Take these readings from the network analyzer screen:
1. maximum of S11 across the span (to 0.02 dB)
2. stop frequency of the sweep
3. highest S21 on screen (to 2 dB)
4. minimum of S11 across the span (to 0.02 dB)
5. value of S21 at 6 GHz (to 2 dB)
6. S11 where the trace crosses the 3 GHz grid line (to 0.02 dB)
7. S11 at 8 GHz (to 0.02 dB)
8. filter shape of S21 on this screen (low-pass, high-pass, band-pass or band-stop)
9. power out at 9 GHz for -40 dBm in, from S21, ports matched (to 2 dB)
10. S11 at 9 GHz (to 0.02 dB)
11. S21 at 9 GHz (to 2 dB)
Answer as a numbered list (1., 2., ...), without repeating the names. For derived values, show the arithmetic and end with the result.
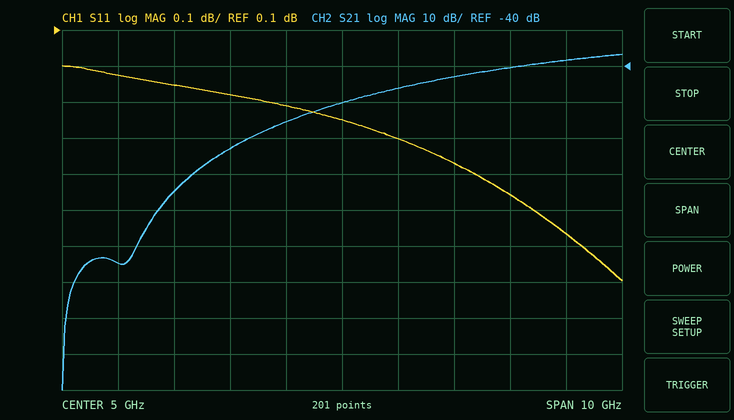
1. 0.00 dB
2. 10 GHz
3. -36 dB
4. -0.60 dB
5. -46 dB
6. -0.08 dB
7. -0.36 dB
8. high-pass
9. -40 dBm + (-38 dB) = -78 dBm
10. -0.46 dB
11. -38 dB
